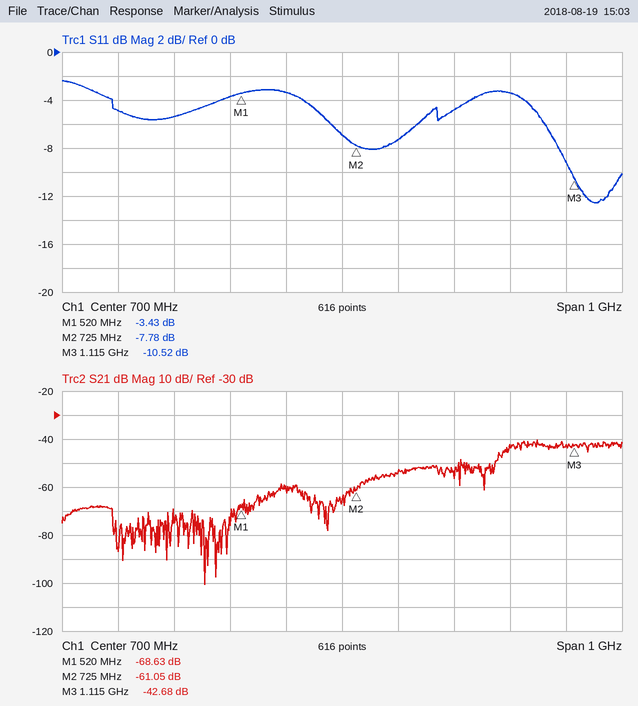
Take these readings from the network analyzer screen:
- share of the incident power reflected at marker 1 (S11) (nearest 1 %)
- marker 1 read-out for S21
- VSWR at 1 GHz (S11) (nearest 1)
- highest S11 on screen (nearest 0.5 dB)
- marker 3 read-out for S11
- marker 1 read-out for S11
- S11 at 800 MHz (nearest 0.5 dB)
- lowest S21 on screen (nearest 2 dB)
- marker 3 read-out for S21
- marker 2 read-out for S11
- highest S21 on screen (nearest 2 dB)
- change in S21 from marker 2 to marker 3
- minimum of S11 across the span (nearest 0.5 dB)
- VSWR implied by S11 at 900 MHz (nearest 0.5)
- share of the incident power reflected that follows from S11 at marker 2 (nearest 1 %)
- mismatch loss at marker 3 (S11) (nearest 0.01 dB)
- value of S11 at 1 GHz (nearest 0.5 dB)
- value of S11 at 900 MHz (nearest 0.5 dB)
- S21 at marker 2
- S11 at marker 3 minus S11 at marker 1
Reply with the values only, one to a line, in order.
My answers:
45 %
-68.63 dB
5
-2.5 dB
-10.52 dB
-3.43 dB
-7.5 dB
-100 dB
-42.68 dB
-7.78 dB
-40 dB
18.37 dB
-12.5 dB
3.5
17 %
0.40 dB
-3.5 dB
-5.0 dB
-61.05 dB
-7.09 dB
